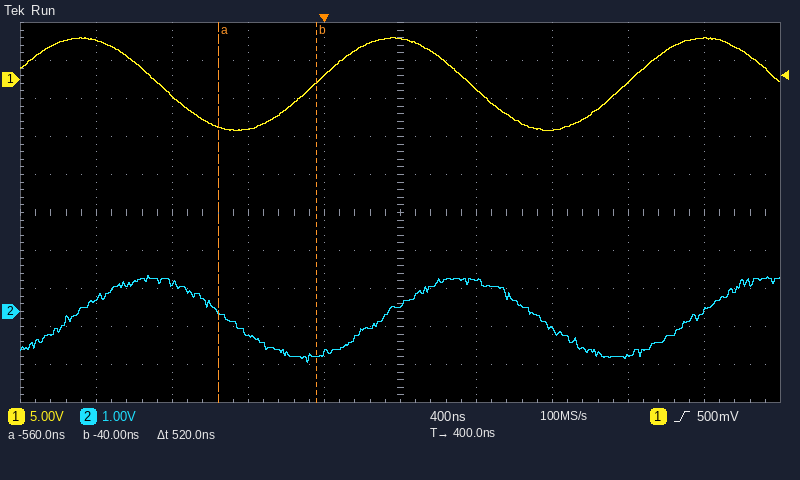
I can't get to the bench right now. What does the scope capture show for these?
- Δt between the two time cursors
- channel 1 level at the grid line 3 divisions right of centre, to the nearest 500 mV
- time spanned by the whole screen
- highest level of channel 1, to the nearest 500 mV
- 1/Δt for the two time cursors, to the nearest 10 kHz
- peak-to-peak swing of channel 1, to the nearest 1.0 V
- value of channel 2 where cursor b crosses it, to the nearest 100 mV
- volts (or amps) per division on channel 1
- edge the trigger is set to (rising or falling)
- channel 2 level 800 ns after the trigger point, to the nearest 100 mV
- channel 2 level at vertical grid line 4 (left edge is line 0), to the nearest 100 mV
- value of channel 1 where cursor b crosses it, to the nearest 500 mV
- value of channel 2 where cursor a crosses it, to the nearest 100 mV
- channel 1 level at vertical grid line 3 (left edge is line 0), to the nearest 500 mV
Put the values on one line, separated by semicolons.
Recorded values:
520 ns; -500 mV; 4 µs; 5.5 V; 1.92 MHz; 12.0 V; -1.2 V; 5 V; rising; 800 mV; -1.1 V; -500 mV; 0.0 V; -6.5 V
